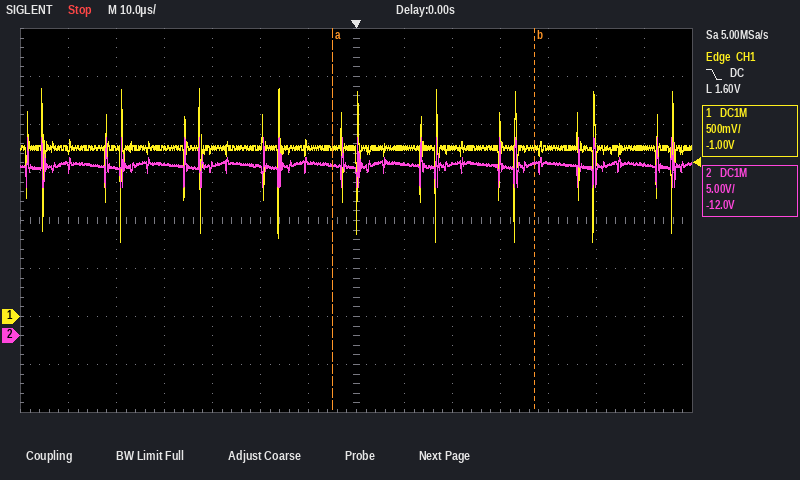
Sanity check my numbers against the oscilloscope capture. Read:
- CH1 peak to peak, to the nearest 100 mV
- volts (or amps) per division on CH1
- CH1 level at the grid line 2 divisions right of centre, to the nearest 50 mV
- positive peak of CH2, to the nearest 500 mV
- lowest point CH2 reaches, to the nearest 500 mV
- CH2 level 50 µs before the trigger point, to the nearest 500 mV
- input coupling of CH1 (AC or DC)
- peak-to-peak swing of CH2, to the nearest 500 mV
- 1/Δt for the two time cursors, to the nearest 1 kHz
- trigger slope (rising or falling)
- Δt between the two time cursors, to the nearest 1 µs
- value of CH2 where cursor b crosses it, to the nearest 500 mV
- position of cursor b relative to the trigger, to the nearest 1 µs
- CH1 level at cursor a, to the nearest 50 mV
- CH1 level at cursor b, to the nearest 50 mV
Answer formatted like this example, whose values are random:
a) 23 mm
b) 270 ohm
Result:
a) 1.60 V
b) 500 mV
c) 1.75 V
d) 20.5 V
e) 15.5 V
f) 17.5 V
g) DC
h) 5.0 V
i) 24 kHz
j) falling
k) 42 µs
l) 18.0 V
m) +37 µs
n) 1.75 V
o) 1.75 V
